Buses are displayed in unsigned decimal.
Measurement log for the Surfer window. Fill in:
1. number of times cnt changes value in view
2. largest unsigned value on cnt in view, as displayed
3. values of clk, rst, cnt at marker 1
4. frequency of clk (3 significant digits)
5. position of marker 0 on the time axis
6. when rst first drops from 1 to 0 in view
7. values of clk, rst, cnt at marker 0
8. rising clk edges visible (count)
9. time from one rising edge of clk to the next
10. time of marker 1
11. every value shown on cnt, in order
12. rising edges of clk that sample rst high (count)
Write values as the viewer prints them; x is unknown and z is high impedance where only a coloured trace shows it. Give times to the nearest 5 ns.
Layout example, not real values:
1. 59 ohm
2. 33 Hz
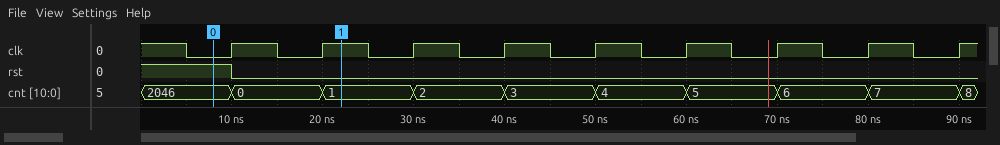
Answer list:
1. 9
2. 2046
3. clk=1, rst=0, cnt=1
4. 100 MHz
5. 10 ns
6. 10 ns
7. clk=0, rst=1, cnt=2046
8. 9
9. 10 ns
10. 20 ns
11. 2046, 0, 1, 2, 3, 4, 5, 6, 7, 8
12. 1
